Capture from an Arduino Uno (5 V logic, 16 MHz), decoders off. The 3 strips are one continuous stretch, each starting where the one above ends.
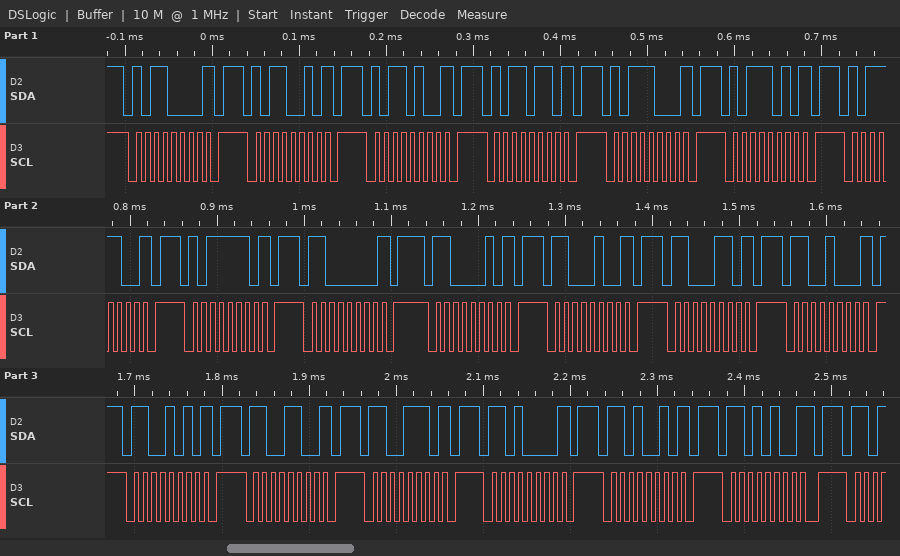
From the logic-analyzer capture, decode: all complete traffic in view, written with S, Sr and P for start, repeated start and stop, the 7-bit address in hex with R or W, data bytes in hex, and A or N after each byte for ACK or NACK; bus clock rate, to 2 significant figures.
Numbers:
S 58W N P S 59W N P S 5AW N P S 5BW N P S 5CW N P S 5DW N P S 5EW N P S 5FW N P S 60W N P S 61W N P S 62W N P S 63W N P S 64W N P S 65W N P S 66W N P S 67W N P S 68W N P S 69W N P S 6AW N P
100 kHz
